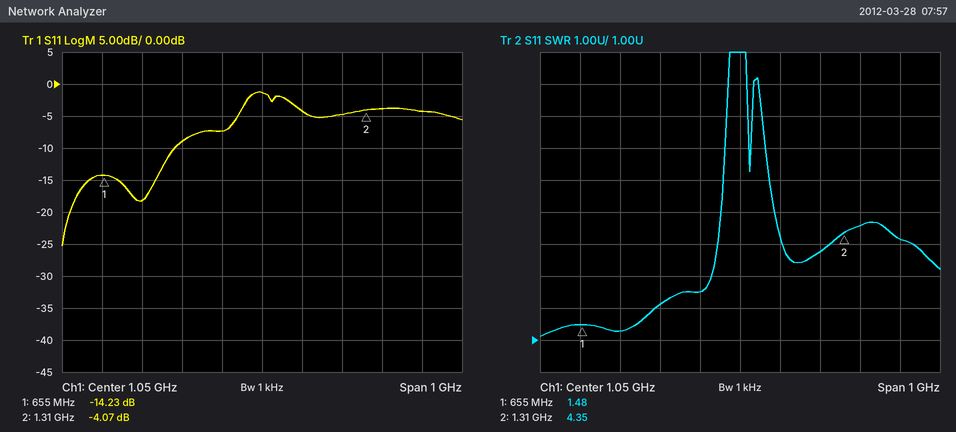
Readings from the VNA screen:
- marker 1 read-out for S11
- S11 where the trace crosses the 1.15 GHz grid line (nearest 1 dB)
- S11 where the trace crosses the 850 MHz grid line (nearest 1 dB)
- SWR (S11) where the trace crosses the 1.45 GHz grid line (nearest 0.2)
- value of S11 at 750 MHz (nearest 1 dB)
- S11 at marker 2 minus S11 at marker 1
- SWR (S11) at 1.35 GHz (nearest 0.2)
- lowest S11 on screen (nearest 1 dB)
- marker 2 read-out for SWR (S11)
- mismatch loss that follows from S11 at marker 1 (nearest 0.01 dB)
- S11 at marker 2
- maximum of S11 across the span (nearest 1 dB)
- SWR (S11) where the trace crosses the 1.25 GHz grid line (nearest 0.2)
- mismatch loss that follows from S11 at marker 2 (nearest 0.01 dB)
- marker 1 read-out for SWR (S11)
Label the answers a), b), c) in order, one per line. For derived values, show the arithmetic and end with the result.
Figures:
a) -14.23 dB
b) -4 dB
c) -9 dB
d) 4.2
e) -18 dB
f) -4.07 − (-14.23) = 10.16 dB
g) 4.6
h) -25 dB
i) 4.35
j) −10 log10(1 − 10^(-14.23/10)) ≈ 0.17 dB
k) -4.07 dB
l) -1 dB
m) 3.8
n) −10 log10(1 − 10^(-4.07/10)) ≈ 2.16 dB
o) 1.48
